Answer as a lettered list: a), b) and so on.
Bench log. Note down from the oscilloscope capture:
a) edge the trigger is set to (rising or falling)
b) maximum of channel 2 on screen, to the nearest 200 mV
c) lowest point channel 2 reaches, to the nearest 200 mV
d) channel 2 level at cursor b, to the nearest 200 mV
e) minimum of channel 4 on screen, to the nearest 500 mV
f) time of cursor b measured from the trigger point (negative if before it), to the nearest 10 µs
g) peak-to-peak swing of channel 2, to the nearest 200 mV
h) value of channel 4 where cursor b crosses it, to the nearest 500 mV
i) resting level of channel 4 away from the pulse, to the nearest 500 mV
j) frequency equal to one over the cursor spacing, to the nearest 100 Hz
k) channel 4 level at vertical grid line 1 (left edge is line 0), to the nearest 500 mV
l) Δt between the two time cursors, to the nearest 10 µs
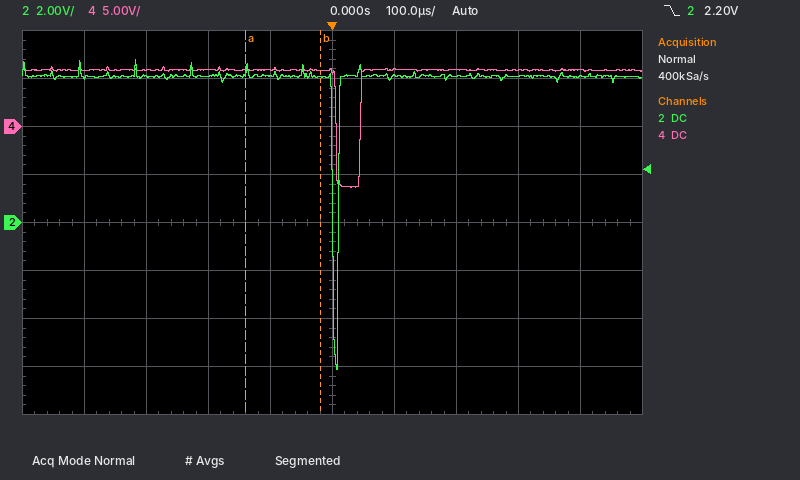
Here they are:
a) falling
b) 6.8 V
c) -6.2 V
d) 6.0 V
e) -6.5 V
f) -20 µs
g) 13.0 V
h) 6.0 V
i) 6.0 V
j) 8.3 kHz
k) 6.0 V
l) 120 µs
